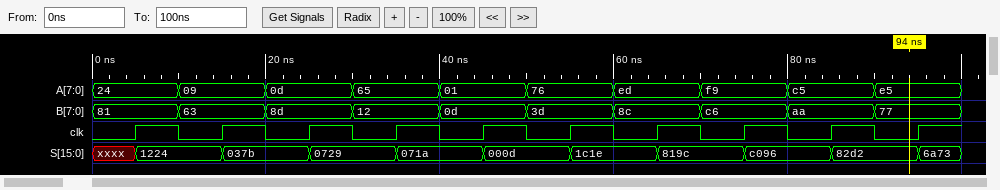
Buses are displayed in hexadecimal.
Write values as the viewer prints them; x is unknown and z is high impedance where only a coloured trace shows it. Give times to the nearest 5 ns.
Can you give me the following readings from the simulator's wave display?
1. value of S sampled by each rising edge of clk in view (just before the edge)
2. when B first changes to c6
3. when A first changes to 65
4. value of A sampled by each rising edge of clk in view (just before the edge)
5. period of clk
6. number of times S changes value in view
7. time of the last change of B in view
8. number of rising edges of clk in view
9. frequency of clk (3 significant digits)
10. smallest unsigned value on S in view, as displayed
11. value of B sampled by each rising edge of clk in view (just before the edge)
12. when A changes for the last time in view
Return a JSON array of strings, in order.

["xxxx, 1224, 037b, 0729, 071a, 000d, 1c1e, 819c, c096, 82d2", "70 ns", "30 ns", "24, 09, 0d, 65, 01, 76, ed, f9, c5, e5", "10 ns", "10", "90 ns", "10", "100 MHz", "000d", "81, 63, 8d, 12, 0d, 3d, 8c, c6, aa, 77", "90 ns"]
